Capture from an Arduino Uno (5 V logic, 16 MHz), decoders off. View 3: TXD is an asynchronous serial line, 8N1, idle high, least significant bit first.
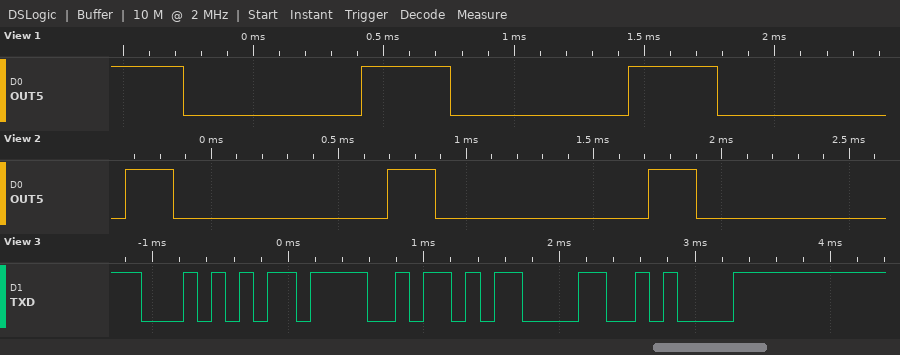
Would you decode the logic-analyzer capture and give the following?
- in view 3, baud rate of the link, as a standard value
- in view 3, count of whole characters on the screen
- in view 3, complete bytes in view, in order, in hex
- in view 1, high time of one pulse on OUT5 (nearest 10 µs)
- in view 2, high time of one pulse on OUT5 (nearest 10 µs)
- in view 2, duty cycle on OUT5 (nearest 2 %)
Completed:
9600 baud
4
54 4F 0D 0A
340 µs
190 µs
18 %
